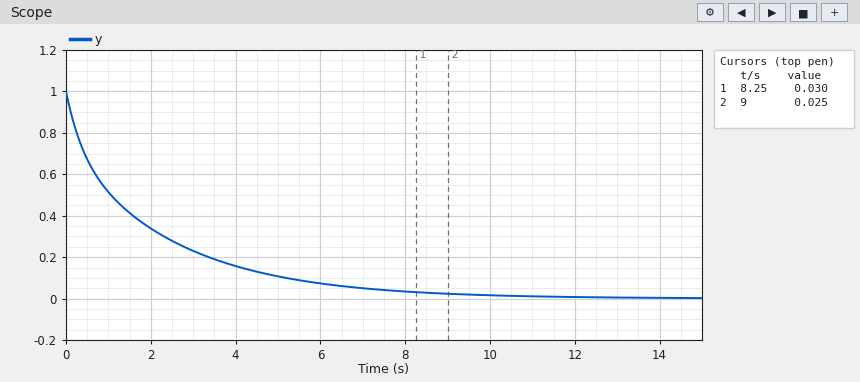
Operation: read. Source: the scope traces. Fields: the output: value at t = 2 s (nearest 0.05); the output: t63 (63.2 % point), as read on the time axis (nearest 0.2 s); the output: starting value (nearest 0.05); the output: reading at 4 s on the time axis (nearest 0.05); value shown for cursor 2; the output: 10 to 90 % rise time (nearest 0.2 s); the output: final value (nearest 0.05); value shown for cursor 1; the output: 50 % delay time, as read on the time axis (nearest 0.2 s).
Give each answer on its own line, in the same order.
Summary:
0.35
1.8 s
1.00
0.15
0.025
5.0 s
0.00
0.030
1.0 s
